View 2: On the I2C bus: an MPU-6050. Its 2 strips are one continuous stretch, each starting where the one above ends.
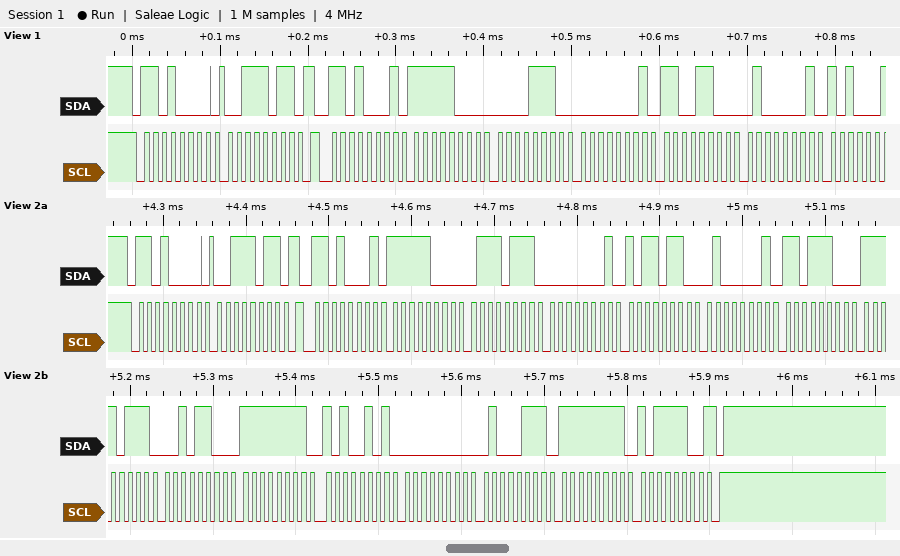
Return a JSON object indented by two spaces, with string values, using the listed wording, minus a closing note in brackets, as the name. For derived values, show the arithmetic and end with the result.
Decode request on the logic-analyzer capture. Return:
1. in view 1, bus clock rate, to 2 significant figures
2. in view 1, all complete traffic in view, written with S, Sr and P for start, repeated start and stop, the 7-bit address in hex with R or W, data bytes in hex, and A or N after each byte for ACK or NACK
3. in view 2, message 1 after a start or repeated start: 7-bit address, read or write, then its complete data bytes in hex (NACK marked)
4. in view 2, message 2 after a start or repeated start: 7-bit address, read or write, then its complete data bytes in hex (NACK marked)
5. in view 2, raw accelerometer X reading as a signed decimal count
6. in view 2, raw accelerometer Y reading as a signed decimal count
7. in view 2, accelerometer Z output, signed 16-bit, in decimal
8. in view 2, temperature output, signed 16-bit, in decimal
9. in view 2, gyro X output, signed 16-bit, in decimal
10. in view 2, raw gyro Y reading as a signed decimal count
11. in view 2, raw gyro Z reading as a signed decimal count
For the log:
{
  "in view 1, bus clock rate, to 2 significant figures": "100 kHz",
  "in view 1, all complete traffic in view, written with S, Sr and P for start, repeated start and stop, the 7-bit address in hex with R or W, data bytes in hex, and A or N after each byte for ACK or NACK": "S 68W A 3B A Sr 68R A F8 A 0E A 01 A CC A 41 A",
  "in view 2, message 1 after a start or repeated start: 7-bit address, read or write, then its complete data bytes in hex": "0x68 write: 3B",
  "in view 2, message 2 after a start or repeated start: 7-bit address, read or write, then its complete data bytes in hex": "0x68 read: F8 77 01 B6 41 DC F7 2C FF A5 00 47 FF BC NACK",
  "in view 2, raw accelerometer X reading as a signed decimal count": "0xF877 = -1929",
  "in view 2, raw accelerometer Y reading as a signed decimal count": "0x01B6 = 438",
  "in view 2, accelerometer Z output, signed 16-bit, in decimal": "0x41DC = 16860",
  "in view 2, temperature output, signed 16-bit, in decimal": "0xF72C = -2260",
  "in view 2, gyro X output, signed 16-bit, in decimal": "0xFFA5 = -91",
  "in view 2, raw gyro Y reading as a signed decimal count": "0x0047 = 71",
  "in view 2, raw gyro Z reading as a signed decimal count": "0xFFBC = -68"
}
